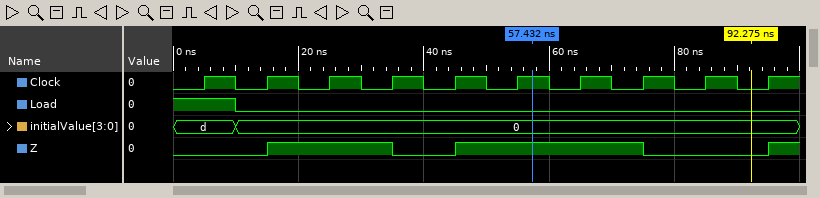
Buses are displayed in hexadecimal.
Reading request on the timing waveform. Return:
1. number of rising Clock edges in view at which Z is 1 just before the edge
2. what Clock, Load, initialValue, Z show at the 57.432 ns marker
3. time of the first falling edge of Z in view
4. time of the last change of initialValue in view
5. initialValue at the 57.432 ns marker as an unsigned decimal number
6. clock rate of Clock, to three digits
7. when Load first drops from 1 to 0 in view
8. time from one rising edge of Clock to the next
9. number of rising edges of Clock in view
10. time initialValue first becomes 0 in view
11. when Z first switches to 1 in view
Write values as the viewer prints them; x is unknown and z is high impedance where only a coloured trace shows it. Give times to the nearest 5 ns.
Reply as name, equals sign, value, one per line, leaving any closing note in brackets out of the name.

number of rising Clock edges in view at which Z is 1 just before the edge = 5
what Clock, Load, initialValue, Z show at the 57.432 ns marker = Clock=1, Load=0, initialValue=0, Z=1
time of the first falling edge of Z in view = 35 ns
time of the last change of initialValue in view = 10 ns
initialValue at the 57.432 ns marker as an unsigned decimal number = 0
clock rate of Clock, to three digits = 100 MHz
when Load first drops from 1 to 0 in view = 10 ns
time from one rising edge of Clock to the next = 10 ns
number of rising edges of Clock in view = 10
time initialValue first becomes 0 in view = 10 ns
when Z first switches to 1 in view = 15 ns
